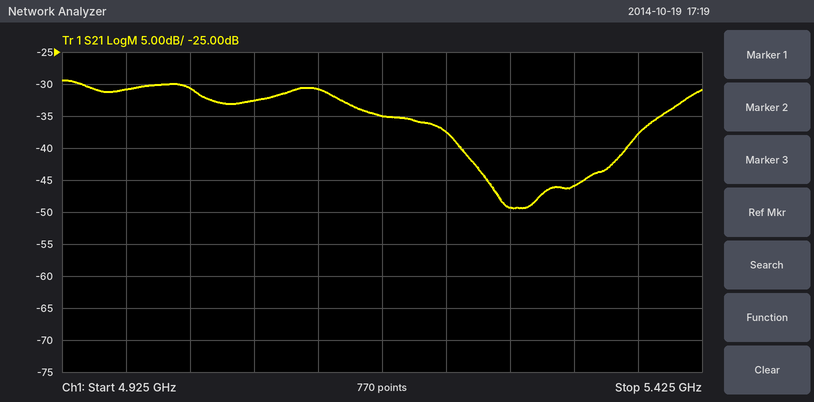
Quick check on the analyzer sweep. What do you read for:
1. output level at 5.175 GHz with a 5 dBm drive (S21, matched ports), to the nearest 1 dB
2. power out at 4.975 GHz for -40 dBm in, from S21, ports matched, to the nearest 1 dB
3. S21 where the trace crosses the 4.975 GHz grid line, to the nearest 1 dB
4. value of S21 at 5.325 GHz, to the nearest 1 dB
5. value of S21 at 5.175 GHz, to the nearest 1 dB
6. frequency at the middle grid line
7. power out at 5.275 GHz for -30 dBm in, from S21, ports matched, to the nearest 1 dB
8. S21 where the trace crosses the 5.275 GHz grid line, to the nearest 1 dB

-30 dBm
-71 dBm
-31 dB
-46 dB
-35 dB
5.175 GHz
-79 dBm
-49 dB
